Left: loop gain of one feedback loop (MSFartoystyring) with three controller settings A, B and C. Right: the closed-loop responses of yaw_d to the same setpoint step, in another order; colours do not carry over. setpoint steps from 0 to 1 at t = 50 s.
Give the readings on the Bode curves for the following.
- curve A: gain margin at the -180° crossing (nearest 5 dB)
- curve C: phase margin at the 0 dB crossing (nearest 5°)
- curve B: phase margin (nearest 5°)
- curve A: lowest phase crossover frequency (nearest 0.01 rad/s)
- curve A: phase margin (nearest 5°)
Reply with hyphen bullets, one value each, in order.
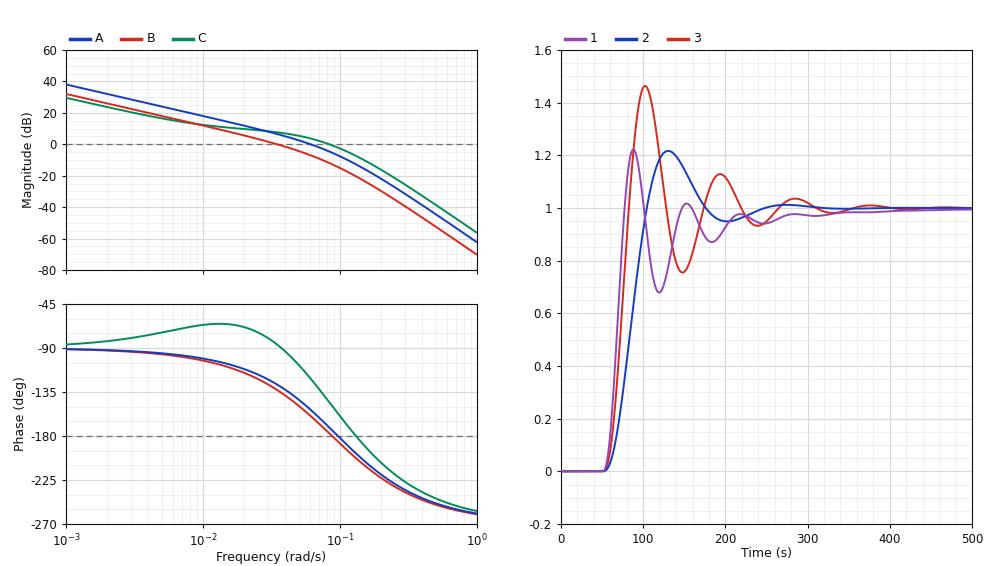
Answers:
- 5 dB
- 35°
- 45°
- 0.10 rad/s
- 25°
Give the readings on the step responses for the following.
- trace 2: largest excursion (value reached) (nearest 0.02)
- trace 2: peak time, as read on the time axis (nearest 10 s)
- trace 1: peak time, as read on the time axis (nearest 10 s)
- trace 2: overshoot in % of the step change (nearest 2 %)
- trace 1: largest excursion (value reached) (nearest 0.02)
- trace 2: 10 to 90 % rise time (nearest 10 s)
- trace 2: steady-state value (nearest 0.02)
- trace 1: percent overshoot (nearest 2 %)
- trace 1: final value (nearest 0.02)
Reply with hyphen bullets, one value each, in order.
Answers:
- 1.22
- 130 s
- 90 s
- 22 %
- 1.22
- 30 s
- 1.00
- 22 %
- 1.00
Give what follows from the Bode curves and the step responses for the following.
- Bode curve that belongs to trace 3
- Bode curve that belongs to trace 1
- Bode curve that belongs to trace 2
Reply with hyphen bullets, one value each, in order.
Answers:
- A
- C
- B
